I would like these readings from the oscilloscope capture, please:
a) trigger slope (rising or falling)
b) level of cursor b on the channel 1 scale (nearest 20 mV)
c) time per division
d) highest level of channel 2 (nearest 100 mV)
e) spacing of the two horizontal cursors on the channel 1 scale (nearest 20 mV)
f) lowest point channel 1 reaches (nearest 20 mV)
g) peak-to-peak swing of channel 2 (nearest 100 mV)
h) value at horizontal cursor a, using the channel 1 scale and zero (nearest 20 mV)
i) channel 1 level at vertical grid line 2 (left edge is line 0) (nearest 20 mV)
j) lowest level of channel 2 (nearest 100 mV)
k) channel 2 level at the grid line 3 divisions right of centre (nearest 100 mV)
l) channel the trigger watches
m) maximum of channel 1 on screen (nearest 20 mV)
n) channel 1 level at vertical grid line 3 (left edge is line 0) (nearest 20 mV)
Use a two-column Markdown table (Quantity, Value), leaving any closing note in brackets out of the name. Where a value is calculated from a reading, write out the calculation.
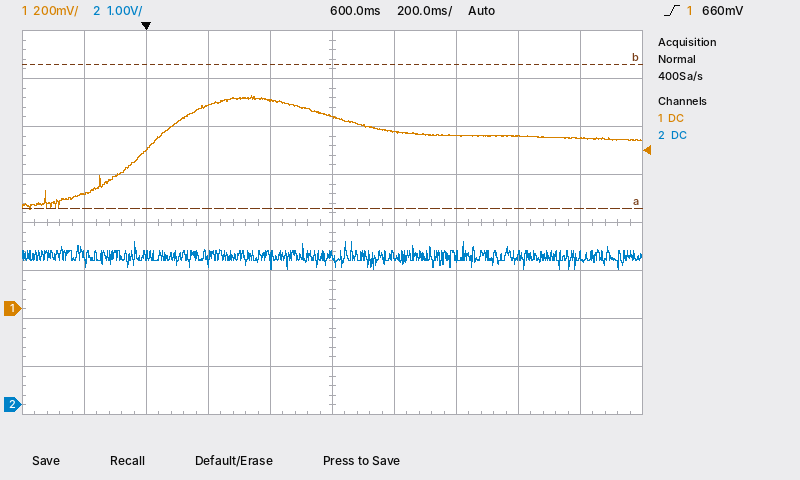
| Quantity | Value |
|---|---|
| trigger slope | rising |
| level of cursor b on the channel 1 scale | 1.02 V |
| time per division | 200 ms |
| highest level of channel 2 | 3.4 V |
| spacing of the two horizontal cursors on the channel 1 scale | 600 mV |
| lowest point channel 1 reaches | 420 mV |
| peak-to-peak swing of channel 2 | 3.4 V − (2.8 V) = 600 mV |
| value at horizontal cursor a, using the channel 1 scale and zero | 420 mV |
| channel 1 level at vertical grid line 2 (left edge is line 0) | 660 mV |
| lowest level of channel 2 | 2.8 V |
| channel 2 level at the grid line 3 divisions right of centre | 3.1 V |
| channel the trigger watches | channel 1 |
| maximum of channel 1 on screen | 880 mV |
| channel 1 level at vertical grid line 3 (left edge is line 0) | 840 mV |
